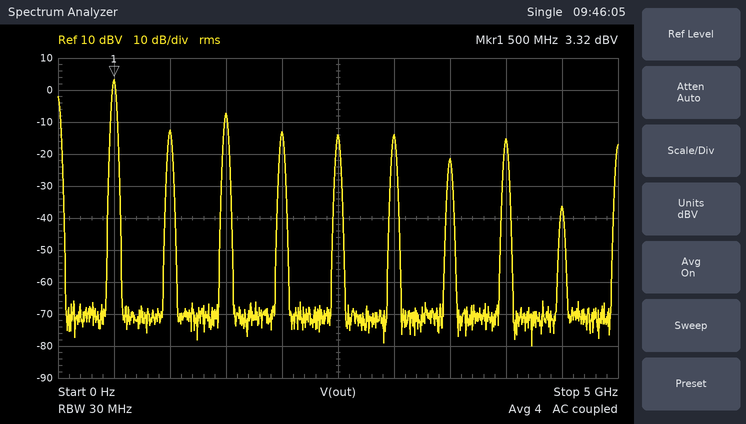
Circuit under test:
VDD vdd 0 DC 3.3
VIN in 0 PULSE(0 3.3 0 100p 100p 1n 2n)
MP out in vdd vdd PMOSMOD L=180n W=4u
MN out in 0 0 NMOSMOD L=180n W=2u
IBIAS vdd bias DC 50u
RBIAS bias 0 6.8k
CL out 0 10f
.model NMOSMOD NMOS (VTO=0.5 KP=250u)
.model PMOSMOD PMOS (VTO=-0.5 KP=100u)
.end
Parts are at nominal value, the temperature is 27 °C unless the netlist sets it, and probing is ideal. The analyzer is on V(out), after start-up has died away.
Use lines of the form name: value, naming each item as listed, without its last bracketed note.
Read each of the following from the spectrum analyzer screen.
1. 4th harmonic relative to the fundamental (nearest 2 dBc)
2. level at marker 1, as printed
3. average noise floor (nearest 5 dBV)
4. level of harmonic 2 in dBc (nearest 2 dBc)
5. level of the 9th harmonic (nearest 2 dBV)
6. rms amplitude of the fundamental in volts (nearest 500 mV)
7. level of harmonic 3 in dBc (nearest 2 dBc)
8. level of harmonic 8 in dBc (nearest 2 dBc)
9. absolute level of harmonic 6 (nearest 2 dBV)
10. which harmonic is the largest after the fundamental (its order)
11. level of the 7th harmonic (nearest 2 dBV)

4th harmonic relative to the fundamental: -16 dBc
level at marker 1, as printed: 3.32 dBV
average noise floor: -70 dBV
level of harmonic 2 in dBc: -16 dBc
level of the 9th harmonic: -36 dBV
rms amplitude of the fundamental in volts: 1.5 V
level of harmonic 3 in dBc: -10 dBc
level of harmonic 8 in dBc: -18 dBc
absolute level of harmonic 6: -14 dBV
which harmonic is the largest after the fundamental: 3
level of the 7th harmonic: -22 dBV
